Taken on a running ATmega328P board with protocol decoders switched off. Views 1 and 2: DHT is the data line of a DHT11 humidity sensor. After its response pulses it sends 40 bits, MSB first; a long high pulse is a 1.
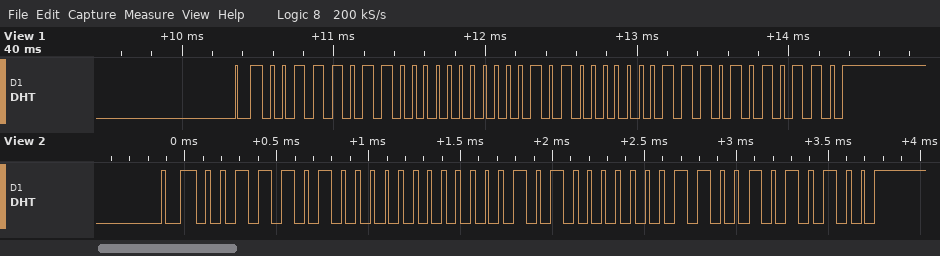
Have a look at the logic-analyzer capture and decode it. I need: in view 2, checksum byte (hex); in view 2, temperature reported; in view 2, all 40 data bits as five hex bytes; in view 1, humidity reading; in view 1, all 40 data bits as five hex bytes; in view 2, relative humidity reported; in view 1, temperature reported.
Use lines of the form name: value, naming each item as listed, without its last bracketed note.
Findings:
in view 2, checksum byte: 0x54
in view 2, temperature reported: 20.6 °C
in view 2, all 40 data bits as five hex bytes: 3A 00 14 06 54
in view 1, humidity reading: 59 %
in view 1, all 40 data bits as five hex bytes: 3B 00 14 07 56
in view 2, relative humidity reported: 58 %
in view 1, temperature reported: 20.7 °C
